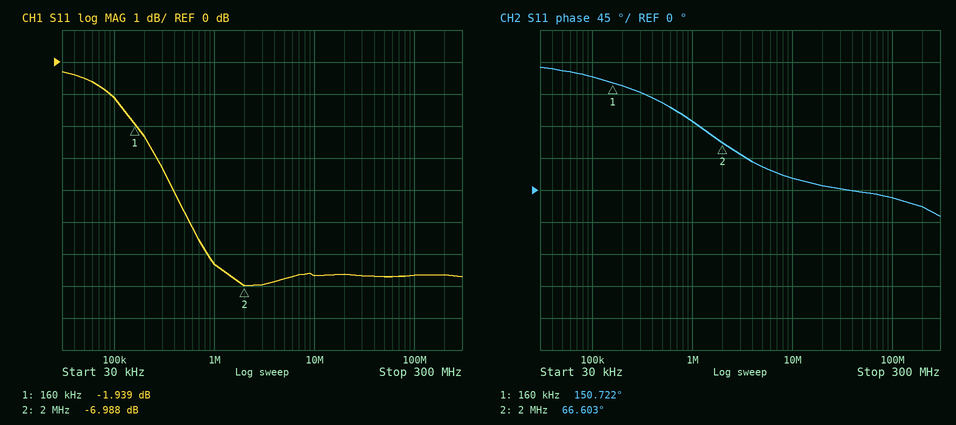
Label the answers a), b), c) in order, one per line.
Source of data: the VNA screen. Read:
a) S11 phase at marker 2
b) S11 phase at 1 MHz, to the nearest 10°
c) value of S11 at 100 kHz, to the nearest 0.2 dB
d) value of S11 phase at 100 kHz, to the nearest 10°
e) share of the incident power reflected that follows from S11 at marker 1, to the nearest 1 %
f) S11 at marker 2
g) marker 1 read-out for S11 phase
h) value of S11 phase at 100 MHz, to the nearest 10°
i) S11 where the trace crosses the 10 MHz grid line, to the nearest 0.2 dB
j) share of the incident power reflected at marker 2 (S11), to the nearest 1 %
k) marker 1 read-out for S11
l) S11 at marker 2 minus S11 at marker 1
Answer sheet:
a) 66.603°
b) 100°
c) -1.2 dB
d) 160°
e) 64 %
f) -6.988 dB
g) 150.722°
h) -10°
i) -6.6 dB
j) 20 %
k) -1.939 dB
l) -5.049 dB
